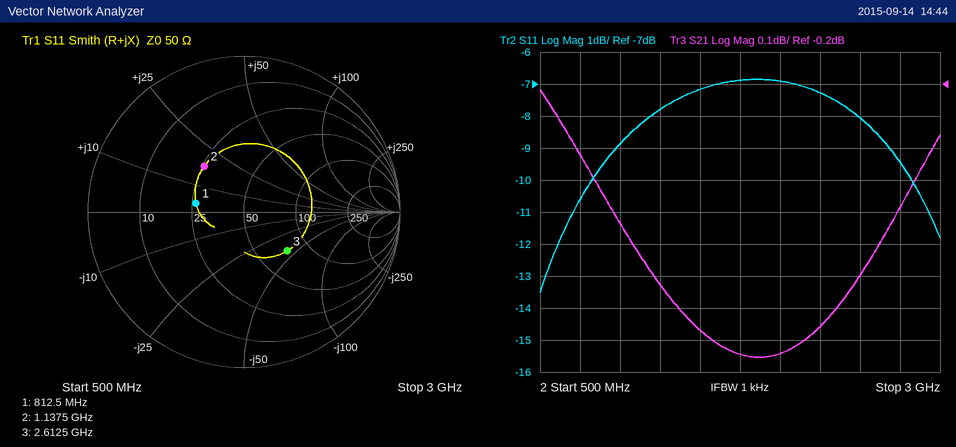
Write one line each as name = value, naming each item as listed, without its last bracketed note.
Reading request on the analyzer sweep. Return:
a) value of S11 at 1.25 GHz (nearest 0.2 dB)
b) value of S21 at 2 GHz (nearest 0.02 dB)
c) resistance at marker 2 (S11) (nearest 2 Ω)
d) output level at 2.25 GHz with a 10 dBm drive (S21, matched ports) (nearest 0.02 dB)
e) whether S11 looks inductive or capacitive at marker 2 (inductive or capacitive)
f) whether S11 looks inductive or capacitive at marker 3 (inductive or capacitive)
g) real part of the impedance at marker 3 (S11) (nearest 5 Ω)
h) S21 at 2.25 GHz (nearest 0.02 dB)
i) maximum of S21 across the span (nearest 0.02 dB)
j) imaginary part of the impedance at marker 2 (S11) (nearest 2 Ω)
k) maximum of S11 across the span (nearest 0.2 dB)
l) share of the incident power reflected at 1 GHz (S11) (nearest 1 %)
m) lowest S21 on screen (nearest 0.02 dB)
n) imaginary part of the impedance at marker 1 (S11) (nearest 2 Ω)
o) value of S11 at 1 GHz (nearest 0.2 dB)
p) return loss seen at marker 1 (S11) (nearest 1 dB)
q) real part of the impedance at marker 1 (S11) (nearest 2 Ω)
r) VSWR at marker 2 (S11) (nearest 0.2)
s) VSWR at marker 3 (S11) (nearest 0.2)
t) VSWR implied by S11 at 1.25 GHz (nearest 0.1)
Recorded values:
value of S11 at 1.25 GHz = -7.8 dB
value of S21 at 2 GHz = -1.04 dB
resistance at marker 2 (S11) = 26 Ω
output level at 2.25 GHz with a 10 dBm drive (S21, matched ports) = 9.04 dBm
whether S11 looks inductive or capacitive at marker 2 = inductive
whether S11 looks inductive or capacitive at marker 3 = capacitive
real part of the impedance at marker 3 (S11) = 75 Ω
S21 at 2.25 GHz = -0.96 dB
maximum of S21 across the span = -0.22 dB
imaginary part of the impedance at marker 2 (S11) = +18 Ω
maximum of S11 across the span = -6.8 dB
share of the incident power reflected at 1 GHz (S11) = 13 %
lowest S21 on screen = -1.06 dB
imaginary part of the impedance at marker 1 (S11) = +4 Ω
value of S11 at 1 GHz = -8.8 dB
return loss seen at marker 1 (S11) = 10 dB
real part of the impedance at marker 1 (S11) = 26 Ω
VSWR at marker 2 (S11) = 2.2
VSWR at marker 3 (S11) = 2.2
VSWR implied by S11 at 1.25 GHz = 2.4
